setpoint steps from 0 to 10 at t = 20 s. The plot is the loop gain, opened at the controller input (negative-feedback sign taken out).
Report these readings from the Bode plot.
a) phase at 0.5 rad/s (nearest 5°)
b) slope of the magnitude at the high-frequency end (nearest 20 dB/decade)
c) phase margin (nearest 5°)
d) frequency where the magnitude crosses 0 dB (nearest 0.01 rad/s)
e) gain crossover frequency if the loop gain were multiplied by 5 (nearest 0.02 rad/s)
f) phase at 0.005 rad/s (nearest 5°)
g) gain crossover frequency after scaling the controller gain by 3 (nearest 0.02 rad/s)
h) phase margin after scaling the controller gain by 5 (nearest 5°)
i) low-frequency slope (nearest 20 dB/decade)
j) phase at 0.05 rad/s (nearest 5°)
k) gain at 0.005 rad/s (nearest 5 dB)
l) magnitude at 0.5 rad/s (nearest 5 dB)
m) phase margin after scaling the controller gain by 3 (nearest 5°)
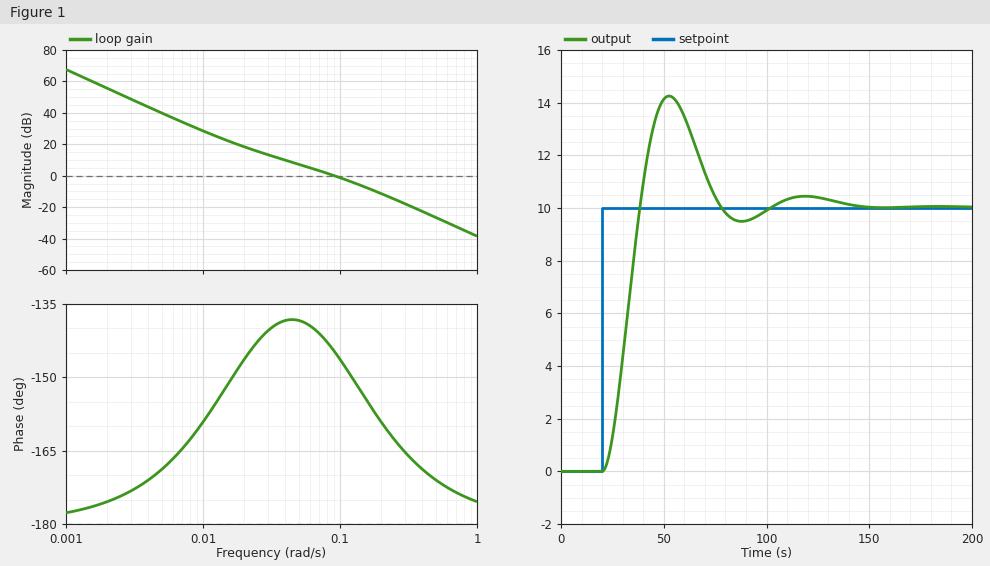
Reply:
-170°
-40 dB/decade
35°
0.09 rad/s
0.24 rad/s
-170°
0.18 rad/s
20°
-40 dB/decade
-140°
40 dB
-25 dB
25°
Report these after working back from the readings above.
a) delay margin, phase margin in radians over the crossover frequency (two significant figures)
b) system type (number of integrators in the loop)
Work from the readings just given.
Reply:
6.8 s
2
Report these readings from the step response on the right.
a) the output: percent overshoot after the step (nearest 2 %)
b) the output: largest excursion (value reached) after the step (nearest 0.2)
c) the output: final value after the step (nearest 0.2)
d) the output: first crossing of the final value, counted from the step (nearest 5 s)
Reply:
42 %
14.2
10.0
20 s
